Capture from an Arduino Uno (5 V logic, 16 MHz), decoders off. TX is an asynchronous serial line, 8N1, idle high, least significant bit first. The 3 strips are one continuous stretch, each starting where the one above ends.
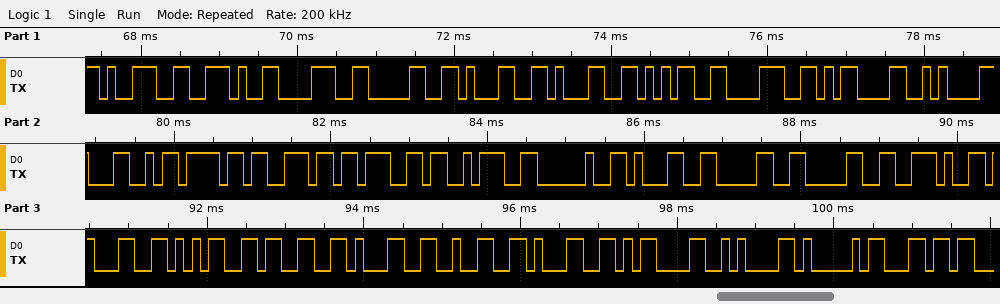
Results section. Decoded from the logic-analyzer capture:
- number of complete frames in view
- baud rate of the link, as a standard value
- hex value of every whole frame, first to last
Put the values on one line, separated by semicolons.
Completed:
30; 9600 baud; 39 2E 38 30 31 31 35 38 0D 0A 4C 6F 6E 67 3A 20 31 30 30 2E 31 35 33 31 32 31 0D 0A 41 6C
